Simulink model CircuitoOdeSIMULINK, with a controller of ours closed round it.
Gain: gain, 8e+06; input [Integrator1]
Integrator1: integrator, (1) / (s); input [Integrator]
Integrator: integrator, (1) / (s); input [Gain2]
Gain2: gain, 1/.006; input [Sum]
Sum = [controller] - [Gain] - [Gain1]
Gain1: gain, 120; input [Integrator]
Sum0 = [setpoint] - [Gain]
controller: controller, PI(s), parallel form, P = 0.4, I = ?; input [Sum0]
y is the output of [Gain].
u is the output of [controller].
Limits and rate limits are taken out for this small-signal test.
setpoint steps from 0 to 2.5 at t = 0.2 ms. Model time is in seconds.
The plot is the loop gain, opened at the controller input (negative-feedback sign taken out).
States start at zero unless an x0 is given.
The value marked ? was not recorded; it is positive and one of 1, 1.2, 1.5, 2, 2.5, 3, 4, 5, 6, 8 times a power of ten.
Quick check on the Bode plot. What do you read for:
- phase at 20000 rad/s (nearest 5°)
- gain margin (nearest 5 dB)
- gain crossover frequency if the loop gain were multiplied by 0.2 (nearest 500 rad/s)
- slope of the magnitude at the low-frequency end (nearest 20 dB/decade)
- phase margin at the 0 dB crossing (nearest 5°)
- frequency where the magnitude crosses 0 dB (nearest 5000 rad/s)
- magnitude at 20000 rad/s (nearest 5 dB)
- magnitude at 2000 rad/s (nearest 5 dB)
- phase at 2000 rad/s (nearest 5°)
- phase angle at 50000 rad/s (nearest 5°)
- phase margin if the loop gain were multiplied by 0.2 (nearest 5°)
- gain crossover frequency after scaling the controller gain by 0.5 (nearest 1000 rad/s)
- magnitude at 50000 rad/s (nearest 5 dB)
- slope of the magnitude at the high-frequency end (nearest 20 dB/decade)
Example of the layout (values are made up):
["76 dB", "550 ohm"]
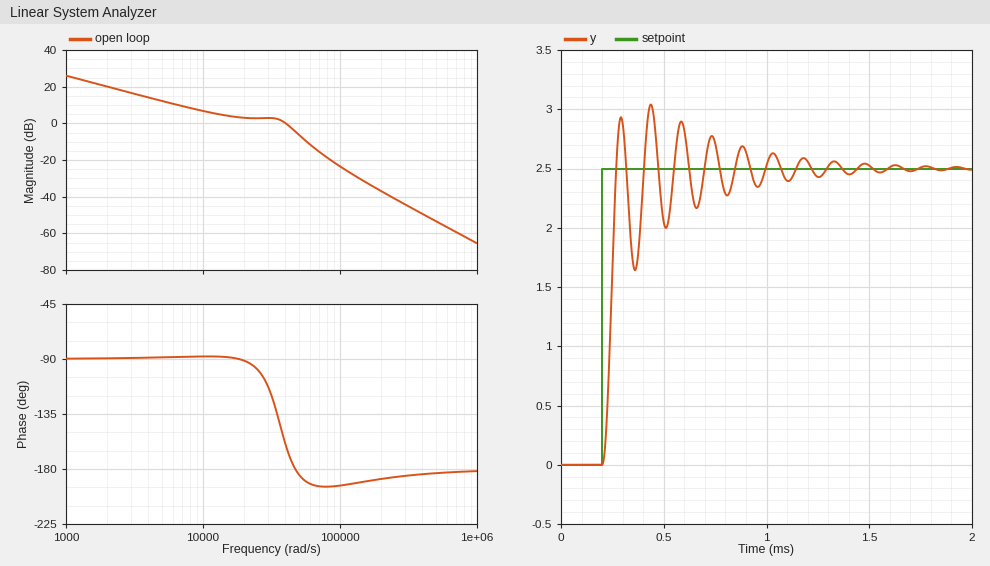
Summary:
["-90°", "5 dB", "4000 rad/s", "-20 dB/decade", "20°", "40000 rad/s", "5 dB", "20 dB", "-90°", "-185°", "90°", "11000 rad/s", "-5 dB", "-40 dB/decade"]
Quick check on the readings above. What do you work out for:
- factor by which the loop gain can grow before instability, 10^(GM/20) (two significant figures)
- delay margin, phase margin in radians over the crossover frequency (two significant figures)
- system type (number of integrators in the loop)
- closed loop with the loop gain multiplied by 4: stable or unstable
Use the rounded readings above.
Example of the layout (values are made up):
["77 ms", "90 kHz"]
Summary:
["1.8", "0.0000087 s", "1", "unstable"]
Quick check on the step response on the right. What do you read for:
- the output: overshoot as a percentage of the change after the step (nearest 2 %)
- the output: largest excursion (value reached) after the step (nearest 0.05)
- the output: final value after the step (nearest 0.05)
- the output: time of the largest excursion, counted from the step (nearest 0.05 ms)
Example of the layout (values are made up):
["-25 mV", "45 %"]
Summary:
["22 %", "3.05", "2.50", "0.25 ms"]
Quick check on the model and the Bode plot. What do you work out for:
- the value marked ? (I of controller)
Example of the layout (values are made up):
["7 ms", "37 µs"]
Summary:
["20000"]
